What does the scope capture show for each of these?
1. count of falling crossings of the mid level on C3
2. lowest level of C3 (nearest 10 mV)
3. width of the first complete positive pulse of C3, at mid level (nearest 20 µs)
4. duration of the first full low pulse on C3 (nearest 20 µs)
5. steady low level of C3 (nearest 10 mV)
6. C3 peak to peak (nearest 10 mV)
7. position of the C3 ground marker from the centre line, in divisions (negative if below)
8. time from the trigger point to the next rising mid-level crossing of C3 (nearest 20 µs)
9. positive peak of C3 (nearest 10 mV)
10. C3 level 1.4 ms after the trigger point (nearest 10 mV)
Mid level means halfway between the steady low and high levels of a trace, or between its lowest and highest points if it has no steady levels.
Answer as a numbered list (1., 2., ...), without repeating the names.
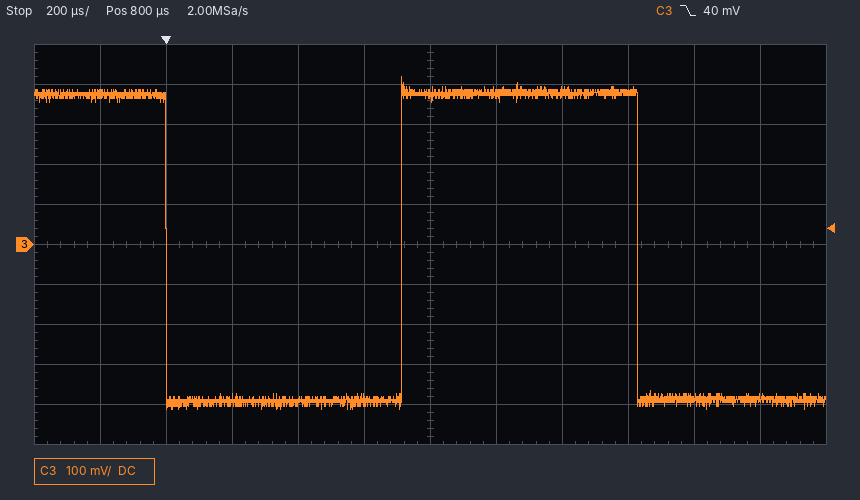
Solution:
1. 2
2. -410 mV
3. 720 µs
4. 720 µs
5. -390 mV
6. 830 mV
7. 0.0 div
8. 720 µs
9. 420 mV
10. 380 mV
